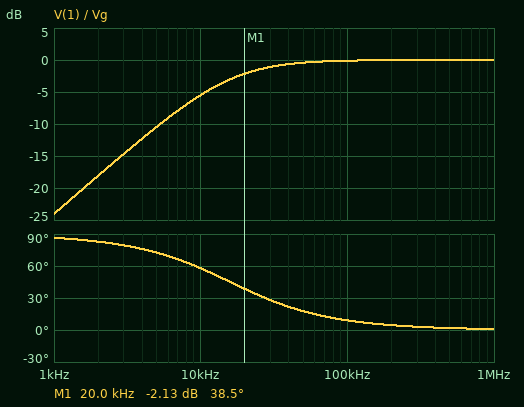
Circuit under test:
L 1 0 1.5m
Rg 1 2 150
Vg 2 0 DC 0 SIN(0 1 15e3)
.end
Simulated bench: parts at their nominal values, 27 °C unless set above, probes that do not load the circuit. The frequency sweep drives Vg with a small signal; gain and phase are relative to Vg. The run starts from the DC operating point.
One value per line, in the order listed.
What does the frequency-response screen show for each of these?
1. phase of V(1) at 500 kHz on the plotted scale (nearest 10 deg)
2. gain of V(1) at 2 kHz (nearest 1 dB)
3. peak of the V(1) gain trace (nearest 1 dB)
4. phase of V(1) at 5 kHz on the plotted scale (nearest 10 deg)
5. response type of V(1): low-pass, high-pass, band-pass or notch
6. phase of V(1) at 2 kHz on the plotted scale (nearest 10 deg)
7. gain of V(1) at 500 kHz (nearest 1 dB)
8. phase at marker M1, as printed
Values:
0 deg
-18 dB
0 dB
70 deg
high-pass
80 deg
0 dB
38.5 deg
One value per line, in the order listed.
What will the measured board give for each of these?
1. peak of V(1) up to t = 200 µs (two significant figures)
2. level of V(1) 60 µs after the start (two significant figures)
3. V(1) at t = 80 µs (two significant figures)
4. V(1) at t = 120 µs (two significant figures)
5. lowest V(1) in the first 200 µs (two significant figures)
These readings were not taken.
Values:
690 mV
130 mV
600 mV
-290 mV
-690 mV
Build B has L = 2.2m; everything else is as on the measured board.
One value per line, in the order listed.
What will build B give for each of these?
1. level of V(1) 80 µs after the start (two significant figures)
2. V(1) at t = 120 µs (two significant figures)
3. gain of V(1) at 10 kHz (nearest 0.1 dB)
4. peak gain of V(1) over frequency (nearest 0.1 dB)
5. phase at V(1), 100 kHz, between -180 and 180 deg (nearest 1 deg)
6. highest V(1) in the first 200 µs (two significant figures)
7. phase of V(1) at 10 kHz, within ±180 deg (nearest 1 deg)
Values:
770 mV
-480 mV
-3.4 dB
0 dB
6 deg
810 mV
47 deg
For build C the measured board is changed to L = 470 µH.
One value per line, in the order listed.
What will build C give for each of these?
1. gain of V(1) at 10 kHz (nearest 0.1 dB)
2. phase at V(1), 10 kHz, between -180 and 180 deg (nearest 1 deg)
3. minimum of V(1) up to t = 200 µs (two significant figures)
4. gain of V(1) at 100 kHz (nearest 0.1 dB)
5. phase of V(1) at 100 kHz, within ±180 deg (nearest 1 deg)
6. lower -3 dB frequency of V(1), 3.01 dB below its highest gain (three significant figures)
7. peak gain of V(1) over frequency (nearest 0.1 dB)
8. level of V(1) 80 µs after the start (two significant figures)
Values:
-14.3 dB
79 deg
-280 mV
-1.0 dB
27 deg
50.8 kHz
0 dB
160 mV
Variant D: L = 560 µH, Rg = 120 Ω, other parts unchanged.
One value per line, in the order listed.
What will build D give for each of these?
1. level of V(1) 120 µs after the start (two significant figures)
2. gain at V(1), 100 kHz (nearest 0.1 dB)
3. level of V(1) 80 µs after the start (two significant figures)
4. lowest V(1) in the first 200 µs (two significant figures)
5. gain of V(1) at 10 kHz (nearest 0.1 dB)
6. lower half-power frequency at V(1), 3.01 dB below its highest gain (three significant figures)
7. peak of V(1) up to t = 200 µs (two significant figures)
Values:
-40 mV
-0.5 dB
270 mV
-400 mV
-11.0 dB
34.1 kHz
400 mV
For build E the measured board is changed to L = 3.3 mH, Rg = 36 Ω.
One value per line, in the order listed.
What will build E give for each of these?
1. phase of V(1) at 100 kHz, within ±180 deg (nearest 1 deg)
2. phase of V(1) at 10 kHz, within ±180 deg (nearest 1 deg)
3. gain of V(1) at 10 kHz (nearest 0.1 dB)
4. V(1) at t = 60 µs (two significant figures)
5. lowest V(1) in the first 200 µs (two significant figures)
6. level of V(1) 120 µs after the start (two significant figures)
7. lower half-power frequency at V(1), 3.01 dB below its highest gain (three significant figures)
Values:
1 deg
10 deg
-0.1 dB
-550 mV
-1.1 V
-930 mV
1.74 kHz
